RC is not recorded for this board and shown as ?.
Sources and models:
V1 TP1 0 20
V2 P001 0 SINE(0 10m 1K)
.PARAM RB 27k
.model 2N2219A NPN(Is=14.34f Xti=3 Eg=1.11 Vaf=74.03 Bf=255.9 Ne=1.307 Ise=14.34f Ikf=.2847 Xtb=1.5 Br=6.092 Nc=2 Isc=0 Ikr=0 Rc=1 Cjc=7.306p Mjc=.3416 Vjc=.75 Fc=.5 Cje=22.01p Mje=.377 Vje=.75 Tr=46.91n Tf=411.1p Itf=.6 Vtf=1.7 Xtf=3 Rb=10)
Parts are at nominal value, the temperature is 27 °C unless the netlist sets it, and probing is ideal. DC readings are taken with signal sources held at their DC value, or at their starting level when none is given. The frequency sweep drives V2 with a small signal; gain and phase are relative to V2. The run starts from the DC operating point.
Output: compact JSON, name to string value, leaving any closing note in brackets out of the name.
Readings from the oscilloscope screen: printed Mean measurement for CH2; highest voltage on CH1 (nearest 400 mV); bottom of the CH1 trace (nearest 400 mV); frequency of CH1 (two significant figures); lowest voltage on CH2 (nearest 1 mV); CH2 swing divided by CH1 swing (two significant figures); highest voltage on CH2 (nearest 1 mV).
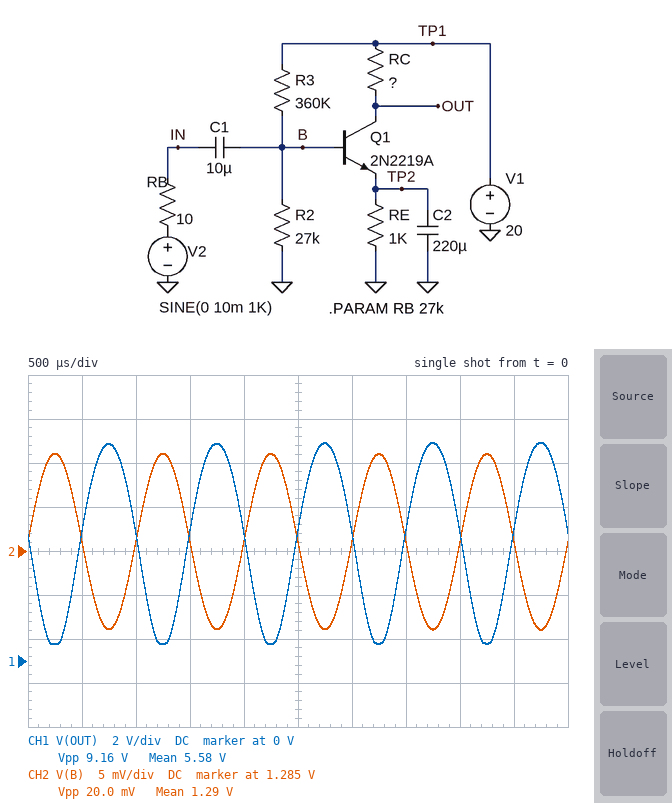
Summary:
{"printed Mean measurement for CH2": "1.29 V", "highest voltage on CH1": "10.0 V", "bottom of the CH1 trace": "800 mV", "frequency of CH1": "1.0 kHz", "lowest voltage on CH2": "1.276 V", "CH2 swing divided by CH1 swing": "0.0022", "highest voltage on CH2": "1.296 V"}
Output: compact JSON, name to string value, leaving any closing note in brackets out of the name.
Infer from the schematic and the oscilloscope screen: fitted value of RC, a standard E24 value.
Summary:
{"fitted value of RC, a standard E24 value": "22 kΩ"}
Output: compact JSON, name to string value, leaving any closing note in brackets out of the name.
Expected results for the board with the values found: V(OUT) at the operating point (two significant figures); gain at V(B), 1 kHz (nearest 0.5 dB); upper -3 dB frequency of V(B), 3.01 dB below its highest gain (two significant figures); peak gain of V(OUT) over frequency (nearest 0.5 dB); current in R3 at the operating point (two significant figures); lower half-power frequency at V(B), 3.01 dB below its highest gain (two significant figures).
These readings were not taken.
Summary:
{"V(OUT) at the operating point": "5.7 V", "gain at V(B), 1 kHz": "0 dB", "upper -3 dB frequency of V(B), 3.01 dB below its highest gain": "230 MHz", "peak gain of V(OUT) over frequency": "53.5 dB", "current in R3 at the operating point": "52 µA", "lower half-power frequency at V(B), 3.01 dB below its highest gain": "890 mHz"}
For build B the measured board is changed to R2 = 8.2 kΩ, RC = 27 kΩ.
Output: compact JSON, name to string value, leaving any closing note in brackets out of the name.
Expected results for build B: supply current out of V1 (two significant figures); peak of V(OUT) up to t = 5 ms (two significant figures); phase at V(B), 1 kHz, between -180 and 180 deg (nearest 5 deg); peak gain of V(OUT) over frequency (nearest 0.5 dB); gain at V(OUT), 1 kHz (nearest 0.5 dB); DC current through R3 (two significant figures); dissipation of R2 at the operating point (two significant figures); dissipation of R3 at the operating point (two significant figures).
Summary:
{"supply current out of V1": "55 µA", "peak of V(OUT) up to t = 5 ms": "20 V", "phase at V(B), 1 kHz, between -180 and 180 deg": "0 deg", "peak gain of V(OUT) over frequency": "0 dB", "gain at V(OUT), 1 kHz": "-5.0 dB", "DC current through R3": "54 µA", "dissipation of R2 at the operating point": "24 µW", "dissipation of R3 at the operating point": "1.1 mW"}
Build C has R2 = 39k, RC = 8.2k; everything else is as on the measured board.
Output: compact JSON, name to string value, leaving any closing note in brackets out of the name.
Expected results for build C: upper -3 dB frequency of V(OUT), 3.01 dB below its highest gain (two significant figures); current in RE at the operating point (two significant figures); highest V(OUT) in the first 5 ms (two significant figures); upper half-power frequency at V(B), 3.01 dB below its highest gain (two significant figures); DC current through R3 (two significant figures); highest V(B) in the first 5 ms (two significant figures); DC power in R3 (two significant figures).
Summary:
{"upper -3 dB frequency of V(OUT), 3.01 dB below its highest gain": "3.9 MHz", "current in RE at the operating point": "1.1 mA", "highest V(OUT) in the first 5 ms": "14 V", "upper half-power frequency at V(B), 3.01 dB below its highest gain": "170 MHz", "DC current through R3": "51 µA", "highest V(B) in the first 5 ms": "1.7 V", "DC power in R3": "930 µW"}
